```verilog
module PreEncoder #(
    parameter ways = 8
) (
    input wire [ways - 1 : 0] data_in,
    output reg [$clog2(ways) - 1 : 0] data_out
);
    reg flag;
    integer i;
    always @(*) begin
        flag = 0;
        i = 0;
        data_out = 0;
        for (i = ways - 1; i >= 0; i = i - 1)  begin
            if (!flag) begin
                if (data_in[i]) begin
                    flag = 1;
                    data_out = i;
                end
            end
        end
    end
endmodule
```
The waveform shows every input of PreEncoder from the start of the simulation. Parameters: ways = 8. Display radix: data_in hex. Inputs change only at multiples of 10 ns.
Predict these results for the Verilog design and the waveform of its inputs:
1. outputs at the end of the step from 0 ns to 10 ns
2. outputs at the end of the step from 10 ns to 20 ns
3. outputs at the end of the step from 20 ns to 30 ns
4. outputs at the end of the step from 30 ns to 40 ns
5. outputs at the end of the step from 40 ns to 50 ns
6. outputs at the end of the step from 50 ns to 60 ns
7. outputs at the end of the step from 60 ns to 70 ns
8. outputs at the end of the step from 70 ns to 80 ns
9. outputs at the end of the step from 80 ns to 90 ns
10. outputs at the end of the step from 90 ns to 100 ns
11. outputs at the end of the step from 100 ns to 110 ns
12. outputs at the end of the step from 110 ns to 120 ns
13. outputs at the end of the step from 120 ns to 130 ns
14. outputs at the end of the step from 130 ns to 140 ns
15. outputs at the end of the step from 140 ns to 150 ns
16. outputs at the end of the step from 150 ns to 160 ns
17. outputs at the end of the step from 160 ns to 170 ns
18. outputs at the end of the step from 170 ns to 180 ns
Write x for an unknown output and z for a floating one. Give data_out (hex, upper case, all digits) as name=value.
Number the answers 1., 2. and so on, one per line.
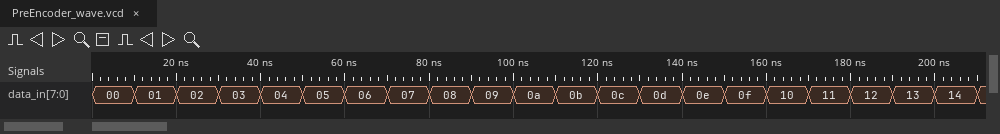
1. data_out=0
2. data_out=0
3. data_out=1
4. data_out=1
5. data_out=2
6. data_out=2
7. data_out=2
8. data_out=2
9. data_out=3
10. data_out=3
11. data_out=3
12. data_out=3
13. data_out=3
14. data_out=3
15. data_out=3
16. data_out=3
17. data_out=4
18. data_out=4
